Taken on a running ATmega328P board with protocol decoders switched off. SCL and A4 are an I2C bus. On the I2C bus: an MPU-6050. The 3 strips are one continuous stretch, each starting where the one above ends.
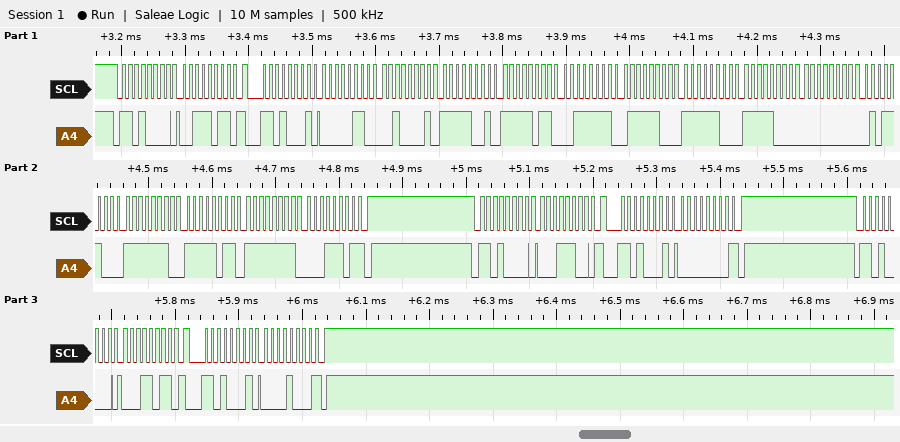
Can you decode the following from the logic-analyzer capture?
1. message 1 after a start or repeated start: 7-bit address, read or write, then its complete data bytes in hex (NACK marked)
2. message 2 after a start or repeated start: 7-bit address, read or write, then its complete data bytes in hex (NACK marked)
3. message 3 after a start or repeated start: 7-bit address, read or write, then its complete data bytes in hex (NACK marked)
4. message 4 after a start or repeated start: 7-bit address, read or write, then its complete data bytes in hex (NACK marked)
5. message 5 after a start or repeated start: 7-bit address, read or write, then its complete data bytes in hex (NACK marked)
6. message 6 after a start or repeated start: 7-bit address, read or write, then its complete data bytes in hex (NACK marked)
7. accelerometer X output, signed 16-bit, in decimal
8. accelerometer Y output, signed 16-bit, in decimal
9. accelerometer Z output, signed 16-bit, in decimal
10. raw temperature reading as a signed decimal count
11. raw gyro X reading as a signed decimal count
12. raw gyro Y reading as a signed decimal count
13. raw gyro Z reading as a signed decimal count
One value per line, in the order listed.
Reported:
0x68 write: 3B
0x68 read: 06 21 F9 FB 3F 7C FC F8 00 5C FE FB FF 1D NACK
0x68 write: 1C
0x68 read: 00 NACK
0x68 write: 1B
0x68 read: 08 NACK
1569
-1541
16252
-776
92
-261
-227
